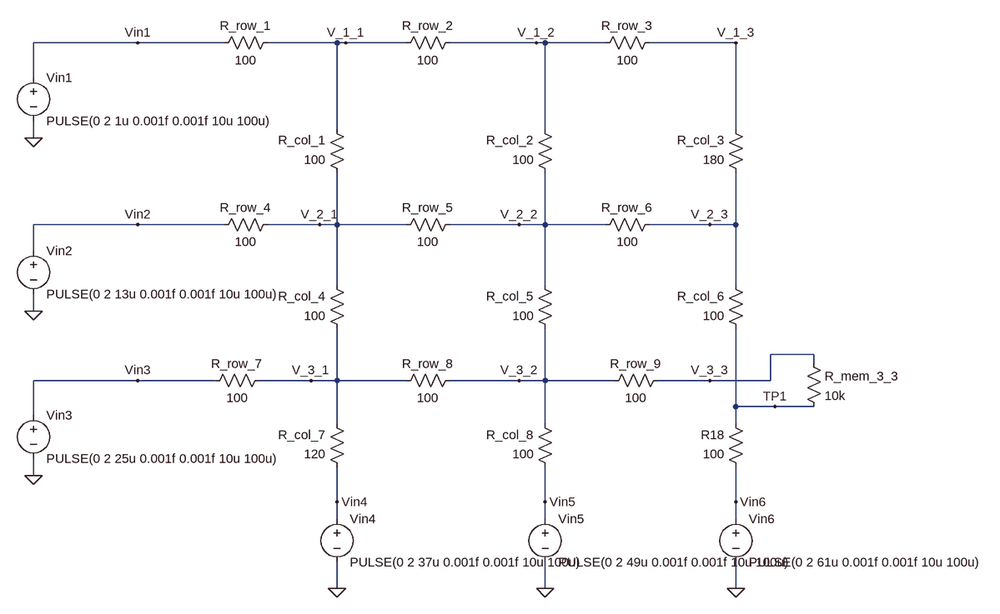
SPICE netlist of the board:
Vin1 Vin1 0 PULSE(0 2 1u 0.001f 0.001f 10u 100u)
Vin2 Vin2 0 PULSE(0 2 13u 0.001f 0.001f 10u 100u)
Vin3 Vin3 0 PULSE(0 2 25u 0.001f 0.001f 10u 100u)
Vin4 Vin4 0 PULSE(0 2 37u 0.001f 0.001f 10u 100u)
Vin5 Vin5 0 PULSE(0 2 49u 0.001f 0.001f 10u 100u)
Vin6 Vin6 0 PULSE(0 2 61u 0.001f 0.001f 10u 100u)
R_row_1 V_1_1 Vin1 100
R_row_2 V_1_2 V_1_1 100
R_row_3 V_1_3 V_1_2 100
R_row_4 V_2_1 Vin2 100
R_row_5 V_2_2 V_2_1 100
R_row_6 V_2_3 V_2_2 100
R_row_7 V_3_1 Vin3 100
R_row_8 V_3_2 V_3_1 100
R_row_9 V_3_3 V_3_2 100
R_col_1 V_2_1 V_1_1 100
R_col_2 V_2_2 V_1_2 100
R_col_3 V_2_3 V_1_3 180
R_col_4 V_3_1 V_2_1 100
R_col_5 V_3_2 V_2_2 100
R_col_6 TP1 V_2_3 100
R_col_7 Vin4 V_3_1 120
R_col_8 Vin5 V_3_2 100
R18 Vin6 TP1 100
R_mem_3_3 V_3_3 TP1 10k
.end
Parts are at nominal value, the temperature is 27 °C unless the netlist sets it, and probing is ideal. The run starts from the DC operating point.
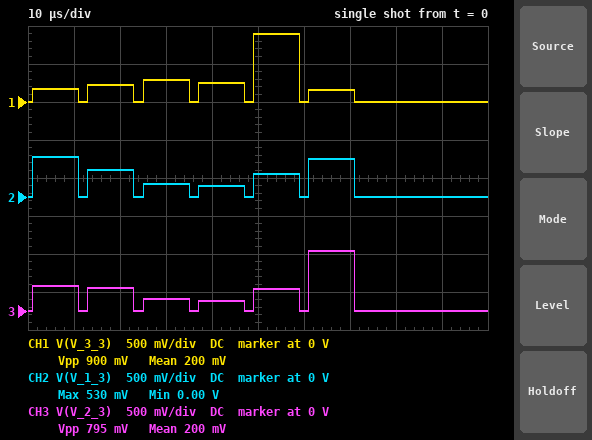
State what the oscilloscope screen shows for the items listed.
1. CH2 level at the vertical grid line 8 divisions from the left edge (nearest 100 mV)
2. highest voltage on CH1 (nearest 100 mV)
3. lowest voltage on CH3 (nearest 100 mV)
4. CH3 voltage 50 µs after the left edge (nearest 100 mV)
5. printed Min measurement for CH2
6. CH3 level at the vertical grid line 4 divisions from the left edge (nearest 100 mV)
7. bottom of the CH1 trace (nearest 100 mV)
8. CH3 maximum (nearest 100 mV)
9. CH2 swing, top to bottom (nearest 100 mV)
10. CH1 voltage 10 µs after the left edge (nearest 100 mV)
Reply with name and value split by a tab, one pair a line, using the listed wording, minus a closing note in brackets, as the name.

CH2 level at the vertical grid line 8 divisions from the left edge	0 V
highest voltage on CH1	900 mV
lowest voltage on CH3	0 V
CH3 voltage 50 µs after the left edge	300 mV
printed Min measurement for CH2	0.00 V
CH3 level at the vertical grid line 4 divisions from the left edge	100 mV
bottom of the CH1 trace	0 V
CH3 maximum	800 mV
CH2 swing, top to bottom	500 mV
CH1 voltage 10 µs after the left edge	200 mV
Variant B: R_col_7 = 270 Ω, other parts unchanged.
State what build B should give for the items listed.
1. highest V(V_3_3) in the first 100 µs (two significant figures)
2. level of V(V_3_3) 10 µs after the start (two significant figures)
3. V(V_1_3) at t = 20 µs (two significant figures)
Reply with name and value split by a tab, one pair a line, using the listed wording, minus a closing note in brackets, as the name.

highest V(V_3_3) in the first 100 µs	920 mV
level of V(V_3_3) 10 µs after the start	190 mV
V(V_1_3) at t = 20 µs	370 mV
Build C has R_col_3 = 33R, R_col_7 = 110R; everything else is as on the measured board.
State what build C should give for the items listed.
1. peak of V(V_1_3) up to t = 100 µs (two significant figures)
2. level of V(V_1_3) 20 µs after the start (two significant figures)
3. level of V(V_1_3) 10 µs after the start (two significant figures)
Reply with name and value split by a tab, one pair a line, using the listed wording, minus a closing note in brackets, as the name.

peak of V(V_1_3) up to t = 100 µs	650 mV
level of V(V_1_3) 20 µs after the start	330 mV
level of V(V_1_3) 10 µs after the start	430 mV
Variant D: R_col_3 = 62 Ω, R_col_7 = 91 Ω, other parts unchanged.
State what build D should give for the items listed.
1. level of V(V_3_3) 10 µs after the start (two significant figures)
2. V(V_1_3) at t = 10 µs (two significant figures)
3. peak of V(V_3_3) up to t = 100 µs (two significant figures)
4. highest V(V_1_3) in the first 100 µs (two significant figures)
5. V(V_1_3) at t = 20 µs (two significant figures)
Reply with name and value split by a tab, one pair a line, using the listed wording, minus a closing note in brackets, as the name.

level of V(V_3_3) 10 µs after the start	170 mV
V(V_1_3) at t = 10 µs	450 mV
peak of V(V_3_3) up to t = 100 µs	890 mV
highest V(V_1_3) in the first 100 µs	610 mV
V(V_1_3) at t = 20 µs	330 mV
